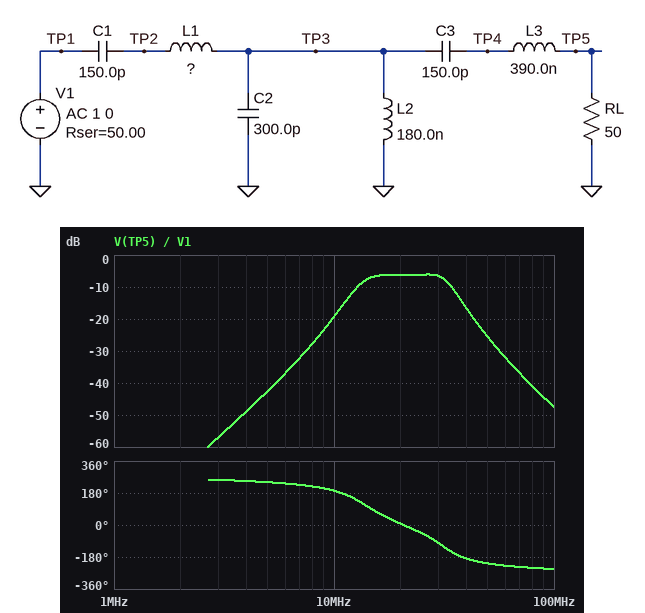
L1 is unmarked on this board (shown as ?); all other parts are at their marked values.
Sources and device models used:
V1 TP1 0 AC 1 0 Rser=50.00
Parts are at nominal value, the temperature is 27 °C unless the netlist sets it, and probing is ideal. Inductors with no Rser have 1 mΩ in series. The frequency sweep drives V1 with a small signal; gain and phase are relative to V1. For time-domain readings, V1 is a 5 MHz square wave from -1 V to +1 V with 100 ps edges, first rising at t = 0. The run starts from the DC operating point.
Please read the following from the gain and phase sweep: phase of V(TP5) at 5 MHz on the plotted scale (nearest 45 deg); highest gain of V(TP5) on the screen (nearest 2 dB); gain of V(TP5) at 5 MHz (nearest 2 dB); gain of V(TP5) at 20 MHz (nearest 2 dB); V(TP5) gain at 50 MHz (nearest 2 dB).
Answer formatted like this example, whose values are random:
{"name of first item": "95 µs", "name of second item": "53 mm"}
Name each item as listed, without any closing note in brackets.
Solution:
{"phase of V(TP5) at 5 MHz on the plotted scale": "225 deg", "highest gain of V(TP5) on the screen": "-6 dB", "gain of V(TP5) at 5 MHz": "-42 dB", "gain of V(TP5) at 20 MHz": "-6 dB", "V(TP5) gain at 50 MHz": "-26 dB"}
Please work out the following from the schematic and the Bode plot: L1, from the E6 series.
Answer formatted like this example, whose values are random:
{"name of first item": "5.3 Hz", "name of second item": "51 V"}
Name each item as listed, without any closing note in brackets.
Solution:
{"L1, from the E6 series": "470 nH"}
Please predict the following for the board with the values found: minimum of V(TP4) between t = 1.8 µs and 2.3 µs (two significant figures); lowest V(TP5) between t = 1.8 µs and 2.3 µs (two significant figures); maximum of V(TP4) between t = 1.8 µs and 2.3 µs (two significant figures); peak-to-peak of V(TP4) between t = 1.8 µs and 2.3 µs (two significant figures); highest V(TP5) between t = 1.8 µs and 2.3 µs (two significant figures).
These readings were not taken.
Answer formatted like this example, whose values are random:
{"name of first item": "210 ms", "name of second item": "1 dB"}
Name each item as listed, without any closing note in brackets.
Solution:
{"minimum of V(TP4) between t = 1.8 µs and 2.3 µs": "-550 mV", "lowest V(TP5) between t = 1.8 µs and 2.3 µs": "-380 mV", "maximum of V(TP4) between t = 1.8 µs and 2.3 µs": "550 mV", "peak-to-peak of V(TP4) between t = 1.8 µs and 2.3 µs": "1.1 V", "highest V(TP5) between t = 1.8 µs and 2.3 µs": "380 mV"}
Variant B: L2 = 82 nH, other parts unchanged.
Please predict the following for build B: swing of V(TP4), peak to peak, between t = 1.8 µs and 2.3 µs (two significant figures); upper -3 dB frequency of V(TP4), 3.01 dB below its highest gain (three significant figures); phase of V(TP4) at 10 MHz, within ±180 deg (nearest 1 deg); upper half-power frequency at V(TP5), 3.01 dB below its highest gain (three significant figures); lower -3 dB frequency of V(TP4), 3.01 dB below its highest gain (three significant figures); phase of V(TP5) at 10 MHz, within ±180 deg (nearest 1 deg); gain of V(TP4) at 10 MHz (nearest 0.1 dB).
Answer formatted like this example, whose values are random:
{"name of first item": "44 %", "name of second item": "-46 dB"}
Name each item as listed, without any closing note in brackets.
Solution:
{"swing of V(TP4), peak to peak, between t = 1.8 µs and 2.3 µs": "810 mV", "upper -3 dB frequency of V(TP4), 3.01 dB below its highest gain": "40.9 MHz", "phase of V(TP4) at 10 MHz, within ±180 deg": "-133 deg", "upper half-power frequency at V(TP5), 3.01 dB below its highest gain": "40.5 MHz", "lower -3 dB frequency of V(TP4), 3.01 dB below its highest gain": "33.6 MHz", "phase of V(TP5) at 10 MHz, within ±180 deg": "-159 deg", "gain of V(TP4) at 10 MHz": "-27.9 dB"}
